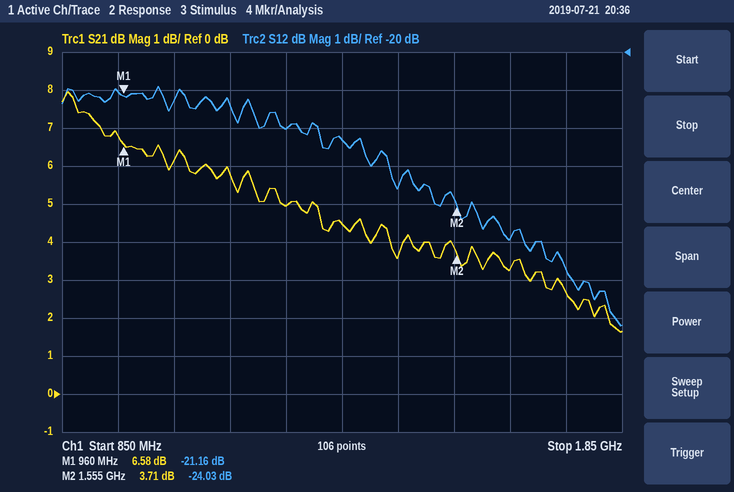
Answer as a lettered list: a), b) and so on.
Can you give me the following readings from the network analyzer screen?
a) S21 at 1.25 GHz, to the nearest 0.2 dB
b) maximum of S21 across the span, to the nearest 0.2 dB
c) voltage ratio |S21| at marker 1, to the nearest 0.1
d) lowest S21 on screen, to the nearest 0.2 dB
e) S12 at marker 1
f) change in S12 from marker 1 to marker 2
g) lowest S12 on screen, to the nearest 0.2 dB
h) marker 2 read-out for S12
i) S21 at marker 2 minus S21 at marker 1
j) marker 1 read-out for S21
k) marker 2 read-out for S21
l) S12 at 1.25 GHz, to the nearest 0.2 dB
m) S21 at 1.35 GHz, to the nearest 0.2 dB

a) 5.0 dB
b) 8.0 dB
c) 2.1
d) 1.6 dB
e) -21.16 dB
f) -2.87 dB
g) -27.2 dB
h) -24.03 dB
i) -2.87 dB
j) 6.58 dB
k) 3.71 dB
l) -22.0 dB
m) 4.4 dB
